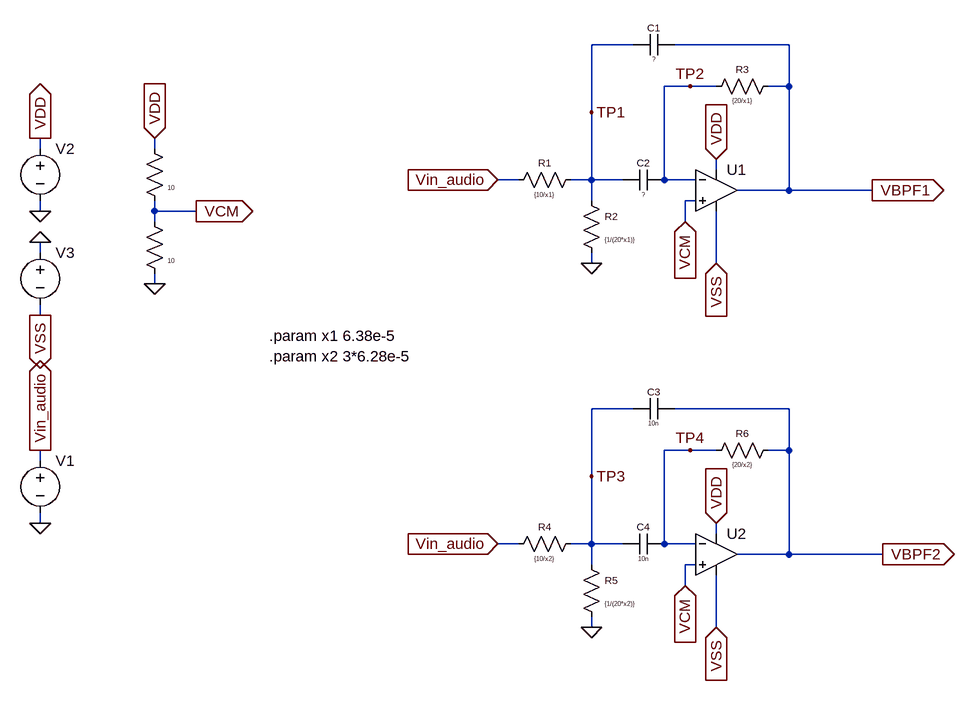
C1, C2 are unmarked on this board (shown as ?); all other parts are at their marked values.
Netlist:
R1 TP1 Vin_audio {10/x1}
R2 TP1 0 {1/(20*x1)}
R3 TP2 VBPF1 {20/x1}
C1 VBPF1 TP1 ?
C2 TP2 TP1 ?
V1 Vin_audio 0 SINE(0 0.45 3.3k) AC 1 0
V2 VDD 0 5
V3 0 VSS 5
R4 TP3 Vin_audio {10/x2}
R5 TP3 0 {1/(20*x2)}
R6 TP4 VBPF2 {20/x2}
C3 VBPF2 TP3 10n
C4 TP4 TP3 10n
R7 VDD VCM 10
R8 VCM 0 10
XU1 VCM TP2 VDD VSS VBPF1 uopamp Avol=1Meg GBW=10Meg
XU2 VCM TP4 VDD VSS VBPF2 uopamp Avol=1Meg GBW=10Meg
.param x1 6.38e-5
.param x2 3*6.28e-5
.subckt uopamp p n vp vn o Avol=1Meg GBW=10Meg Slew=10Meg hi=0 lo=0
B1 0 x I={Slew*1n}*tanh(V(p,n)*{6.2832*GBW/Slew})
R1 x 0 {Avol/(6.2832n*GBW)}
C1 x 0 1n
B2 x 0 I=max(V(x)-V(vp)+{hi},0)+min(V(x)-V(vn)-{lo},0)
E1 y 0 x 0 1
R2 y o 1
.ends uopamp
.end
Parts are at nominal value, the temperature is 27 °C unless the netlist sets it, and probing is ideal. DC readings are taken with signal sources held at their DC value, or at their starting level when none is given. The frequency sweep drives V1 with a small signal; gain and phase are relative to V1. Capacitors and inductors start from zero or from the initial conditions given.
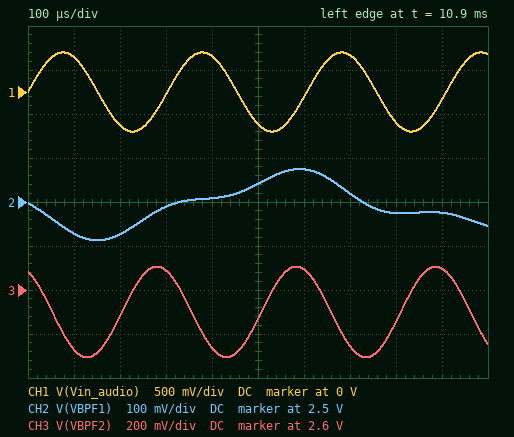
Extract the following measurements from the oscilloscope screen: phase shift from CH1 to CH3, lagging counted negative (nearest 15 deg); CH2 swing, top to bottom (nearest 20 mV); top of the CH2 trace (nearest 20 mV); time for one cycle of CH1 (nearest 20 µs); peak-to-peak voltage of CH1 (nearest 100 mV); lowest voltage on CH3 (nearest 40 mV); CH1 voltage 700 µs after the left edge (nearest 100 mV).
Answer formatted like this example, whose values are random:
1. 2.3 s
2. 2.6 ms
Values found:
1. 120 deg
2. 160 mV
3. 2.58 V
4. 300 µs
5. 900 mV
6. 2.28 V
7. 400 mV
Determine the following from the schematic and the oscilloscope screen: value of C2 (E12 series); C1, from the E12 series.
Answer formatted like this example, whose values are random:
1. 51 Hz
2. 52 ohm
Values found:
1. 8.2 nF
2. 8.2 nF
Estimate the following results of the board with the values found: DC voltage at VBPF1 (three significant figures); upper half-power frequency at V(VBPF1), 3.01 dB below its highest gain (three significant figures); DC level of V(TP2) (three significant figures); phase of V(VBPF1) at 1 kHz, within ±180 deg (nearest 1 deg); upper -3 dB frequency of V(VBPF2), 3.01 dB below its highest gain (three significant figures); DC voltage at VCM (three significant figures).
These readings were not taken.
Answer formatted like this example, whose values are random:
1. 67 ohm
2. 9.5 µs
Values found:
1. 2.50 V
2. 1.30 kHz
3. 2.50 V
4. -103 deg
5. 3.15 kHz
6. 2.50 V
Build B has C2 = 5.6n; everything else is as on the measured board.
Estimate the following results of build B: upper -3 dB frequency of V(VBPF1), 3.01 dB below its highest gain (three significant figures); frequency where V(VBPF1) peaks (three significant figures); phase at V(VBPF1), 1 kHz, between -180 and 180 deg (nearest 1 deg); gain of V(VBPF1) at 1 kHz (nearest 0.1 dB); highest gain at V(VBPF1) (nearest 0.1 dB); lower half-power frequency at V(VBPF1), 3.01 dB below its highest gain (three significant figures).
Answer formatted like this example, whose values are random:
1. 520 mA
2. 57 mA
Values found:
1. 1.58 kHz
2. 1.50 kHz
3. -97 deg
4. -20.2 dB
5. -1.8 dB
6. 1.43 kHz
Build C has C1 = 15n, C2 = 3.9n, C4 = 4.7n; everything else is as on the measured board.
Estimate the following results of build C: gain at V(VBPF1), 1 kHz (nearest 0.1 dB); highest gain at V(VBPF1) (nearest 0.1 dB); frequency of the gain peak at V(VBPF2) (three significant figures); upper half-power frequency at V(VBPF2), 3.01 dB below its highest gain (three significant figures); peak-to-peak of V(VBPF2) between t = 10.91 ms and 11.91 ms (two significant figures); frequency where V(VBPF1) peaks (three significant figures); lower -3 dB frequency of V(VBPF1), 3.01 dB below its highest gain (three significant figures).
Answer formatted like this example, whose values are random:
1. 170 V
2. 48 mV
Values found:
1. -21.3 dB
2. -7.7 dB
3. 4.37 kHz
4. 4.61 kHz
5. 110 mV
6. 1.33 kHz
7. 1.25 kHz
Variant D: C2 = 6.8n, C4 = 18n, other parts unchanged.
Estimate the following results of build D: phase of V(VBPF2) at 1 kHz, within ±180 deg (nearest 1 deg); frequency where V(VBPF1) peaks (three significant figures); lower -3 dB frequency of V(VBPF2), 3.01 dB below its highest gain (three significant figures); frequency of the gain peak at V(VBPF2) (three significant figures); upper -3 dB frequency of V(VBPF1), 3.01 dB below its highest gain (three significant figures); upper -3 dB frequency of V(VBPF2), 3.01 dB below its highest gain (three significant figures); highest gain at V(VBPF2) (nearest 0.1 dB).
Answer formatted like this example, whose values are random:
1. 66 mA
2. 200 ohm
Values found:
1. -93 deg
2. 1.36 kHz
3. 2.12 kHz
4. 2.23 kHz
5. 1.43 kHz
6. 2.35 kHz
7. 2.2 dB
